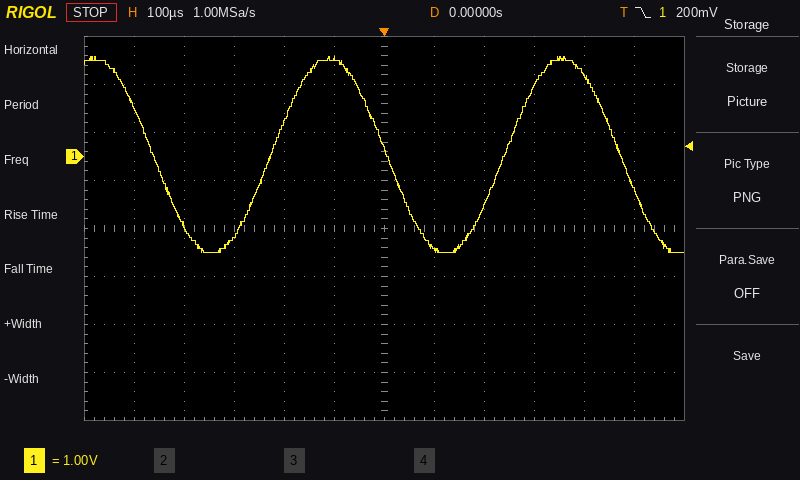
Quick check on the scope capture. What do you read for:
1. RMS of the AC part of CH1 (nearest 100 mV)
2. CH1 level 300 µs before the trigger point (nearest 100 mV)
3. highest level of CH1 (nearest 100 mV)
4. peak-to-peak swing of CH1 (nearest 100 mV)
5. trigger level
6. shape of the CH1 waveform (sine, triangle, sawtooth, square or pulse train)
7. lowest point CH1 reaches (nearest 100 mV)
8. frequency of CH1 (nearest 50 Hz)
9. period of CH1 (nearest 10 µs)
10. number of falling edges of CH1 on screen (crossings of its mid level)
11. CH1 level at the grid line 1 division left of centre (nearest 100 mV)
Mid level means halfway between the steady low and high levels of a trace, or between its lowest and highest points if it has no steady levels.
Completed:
1.4 V
-1.7 V
2.1 V
4.1 V
200 mV
sine
-2.0 V
2.15 kHz
470 µs
3
2.0 V
